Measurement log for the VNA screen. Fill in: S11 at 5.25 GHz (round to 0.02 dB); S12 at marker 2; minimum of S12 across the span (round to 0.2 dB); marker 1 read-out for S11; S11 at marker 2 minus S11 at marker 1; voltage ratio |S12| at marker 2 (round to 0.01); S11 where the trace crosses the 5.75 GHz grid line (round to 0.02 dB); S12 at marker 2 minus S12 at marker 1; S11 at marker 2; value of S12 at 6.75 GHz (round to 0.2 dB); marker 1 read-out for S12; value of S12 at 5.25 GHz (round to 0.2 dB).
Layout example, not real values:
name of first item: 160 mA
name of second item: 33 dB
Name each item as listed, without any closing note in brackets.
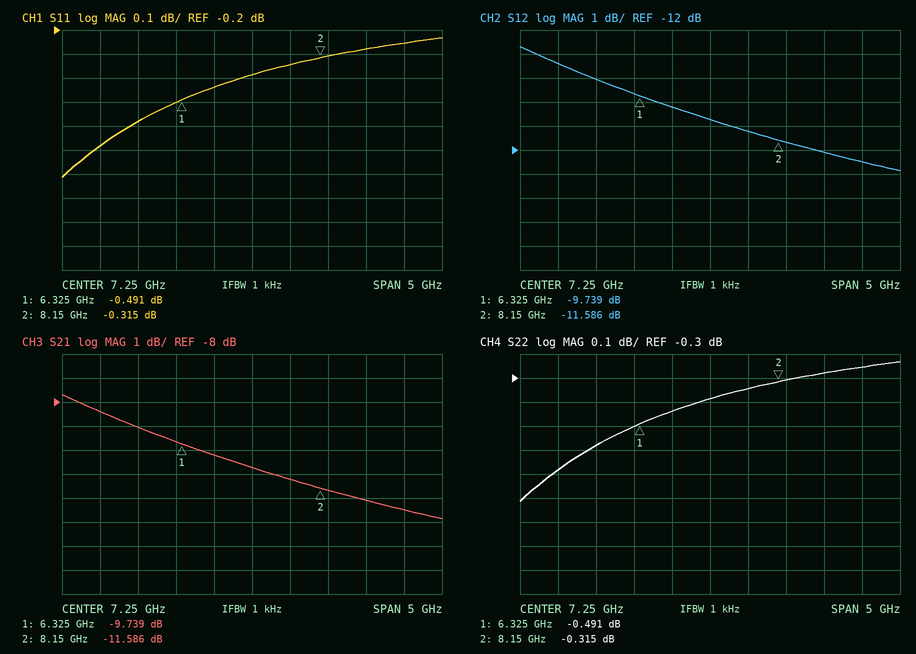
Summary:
S11 at 5.25 GHz: -0.68 dB
S12 at marker 2: -11.586 dB
minimum of S12 across the span: -12.8 dB
marker 1 read-out for S11: -0.491 dB
S11 at marker 2 minus S11 at marker 1: 0.176 dB
voltage ratio |S12| at marker 2: 0.26
S11 where the trace crosses the 5.75 GHz grid line: -0.58 dB
S12 at marker 2 minus S12 at marker 1: -1.847 dB
S11 at marker 2: -0.315 dB
value of S12 at 6.75 GHz: -10.2 dB
marker 1 read-out for S12: -9.739 dB
value of S12 at 5.25 GHz: -8.4 dB
